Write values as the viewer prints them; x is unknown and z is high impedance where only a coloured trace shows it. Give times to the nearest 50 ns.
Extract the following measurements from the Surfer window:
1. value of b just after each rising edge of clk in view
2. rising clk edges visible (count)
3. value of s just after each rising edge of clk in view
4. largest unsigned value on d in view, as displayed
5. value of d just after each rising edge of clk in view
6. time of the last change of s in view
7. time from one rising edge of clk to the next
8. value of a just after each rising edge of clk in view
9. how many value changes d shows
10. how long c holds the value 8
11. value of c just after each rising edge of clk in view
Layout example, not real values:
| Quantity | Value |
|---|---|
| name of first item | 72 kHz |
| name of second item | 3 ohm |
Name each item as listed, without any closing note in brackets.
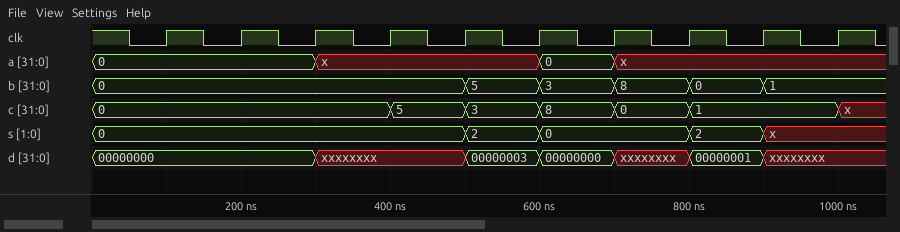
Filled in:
| Quantity | Value |
|---|---|
| value of b just after each rising edge of clk in view | 0, 0, 0, 0, 5, 3, 8, 0, 1, 1 |
| rising clk edges visible | 10 |
| value of s just after each rising edge of clk in view | 0, 0, 0, 0, 2, 0, 0, 2, x, x |
| largest unsigned value on d in view, as displayed | 00000003 |
| value of d just after each rising edge of clk in view | 00000000, 00000000, xxxxxxxx, xxxxxxxx, 00000003, 00000000, xxxxxxxx, 00000001, xxxxxxxx, xxxxxxxx |
| time of the last change of s in view | 900 ns |
| time from one rising edge of clk to the next | 100 ns |
| value of a just after each rising edge of clk in view | 0, 0, x, x, x, 0, x, x, x, x |
| how many value changes d shows | 6 |
| how long c holds the value 8 | 100 ns |
| value of c just after each rising edge of clk in view | 0, 0, 0, 5, 3, 8, 0, 1, 1, x |
